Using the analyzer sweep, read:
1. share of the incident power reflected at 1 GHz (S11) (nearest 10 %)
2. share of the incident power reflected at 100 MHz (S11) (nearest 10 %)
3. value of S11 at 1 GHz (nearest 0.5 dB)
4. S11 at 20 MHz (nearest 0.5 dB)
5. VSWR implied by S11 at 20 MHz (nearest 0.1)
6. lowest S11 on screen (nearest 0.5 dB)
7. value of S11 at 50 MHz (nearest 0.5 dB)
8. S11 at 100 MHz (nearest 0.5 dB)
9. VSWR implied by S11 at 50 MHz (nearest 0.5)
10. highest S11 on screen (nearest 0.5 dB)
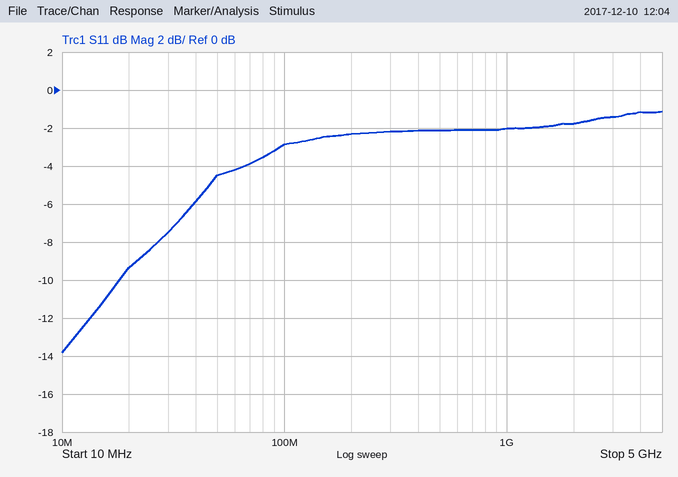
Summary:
60 %
50 %
-2.0 dB
-9.5 dB
2.0
-14.0 dB
-4.5 dB
-3.0 dB
4.0
-1.0 dB
